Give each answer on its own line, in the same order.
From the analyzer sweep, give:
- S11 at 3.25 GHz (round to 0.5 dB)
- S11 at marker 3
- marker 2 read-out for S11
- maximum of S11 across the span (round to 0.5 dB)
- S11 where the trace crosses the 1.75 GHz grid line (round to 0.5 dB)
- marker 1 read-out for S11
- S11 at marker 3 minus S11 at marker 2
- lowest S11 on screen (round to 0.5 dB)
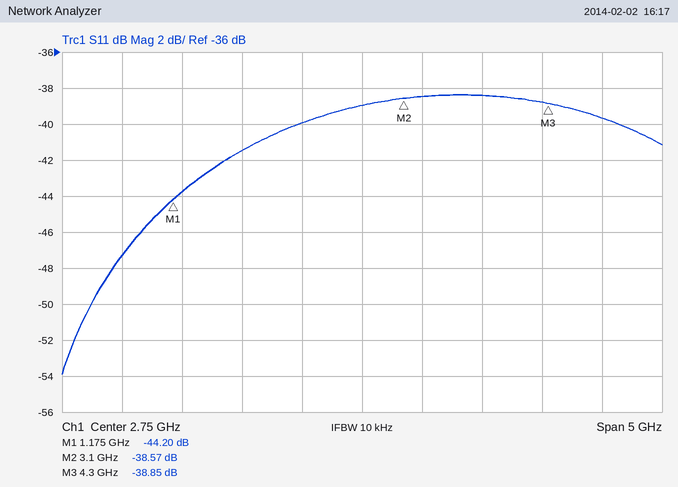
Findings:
-38.5 dB
-38.85 dB
-38.57 dB
-38.5 dB
-41.5 dB
-44.20 dB
-0.28 dB
-54.0 dB
